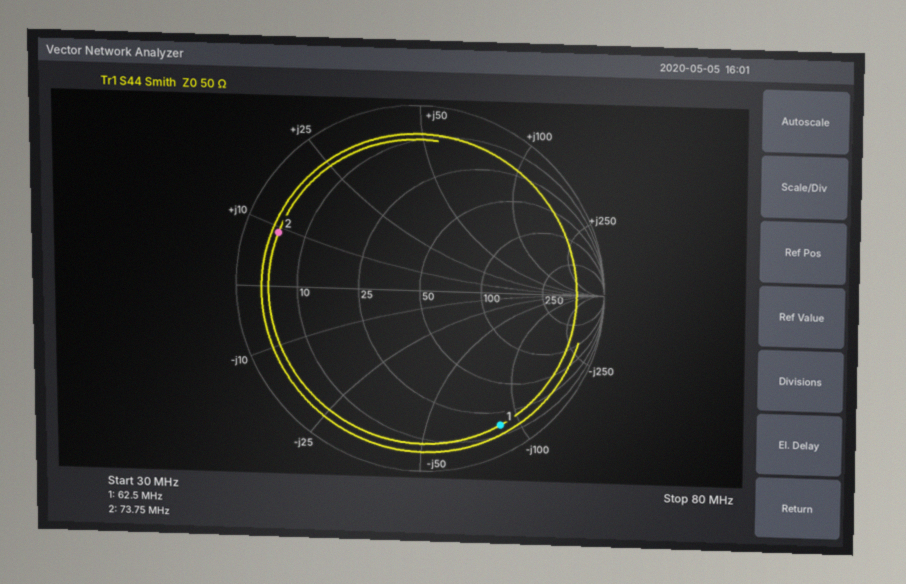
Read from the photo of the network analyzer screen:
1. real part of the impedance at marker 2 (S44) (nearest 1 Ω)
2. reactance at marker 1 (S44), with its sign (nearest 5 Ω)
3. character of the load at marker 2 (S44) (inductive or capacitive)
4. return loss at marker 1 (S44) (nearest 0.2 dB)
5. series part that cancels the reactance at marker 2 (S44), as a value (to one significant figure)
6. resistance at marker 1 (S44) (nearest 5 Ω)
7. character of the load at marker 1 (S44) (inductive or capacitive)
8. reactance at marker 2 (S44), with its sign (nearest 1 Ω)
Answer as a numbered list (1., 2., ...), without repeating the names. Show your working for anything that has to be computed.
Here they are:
1. 5 Ω
2. -85 Ω
3. inductive
4. 1.4 dB
5. C = 1/(2π × 73.75 MHz × 9 Ω) ≈ 240 pF, so 200 pF to one significant figure
6. 15 Ω
7. capacitive
8. +9 Ω
